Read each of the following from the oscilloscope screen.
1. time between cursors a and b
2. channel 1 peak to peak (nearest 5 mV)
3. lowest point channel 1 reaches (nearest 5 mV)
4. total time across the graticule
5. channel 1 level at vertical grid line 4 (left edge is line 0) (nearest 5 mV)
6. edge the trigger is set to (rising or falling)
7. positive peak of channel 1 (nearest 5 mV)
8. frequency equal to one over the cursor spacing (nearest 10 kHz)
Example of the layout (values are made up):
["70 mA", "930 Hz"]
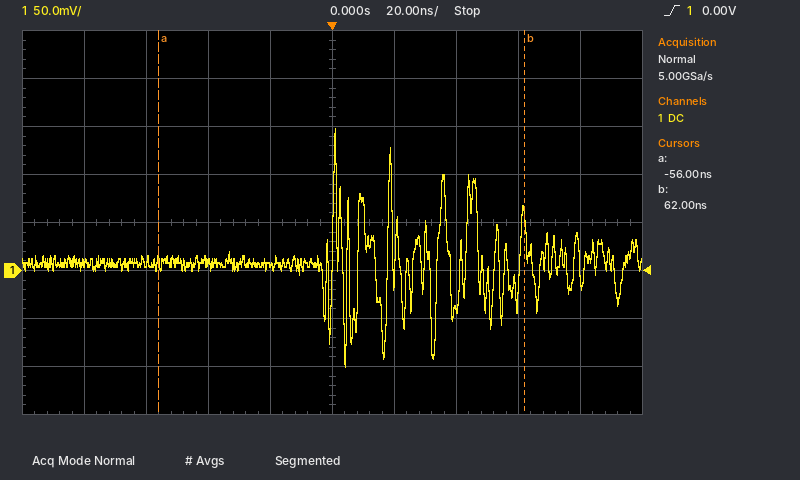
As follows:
["118 ns", "250 mV", "-100 mV", "200 ns", "5 mV", "rising", "150 mV", "8.47 MHz"]
